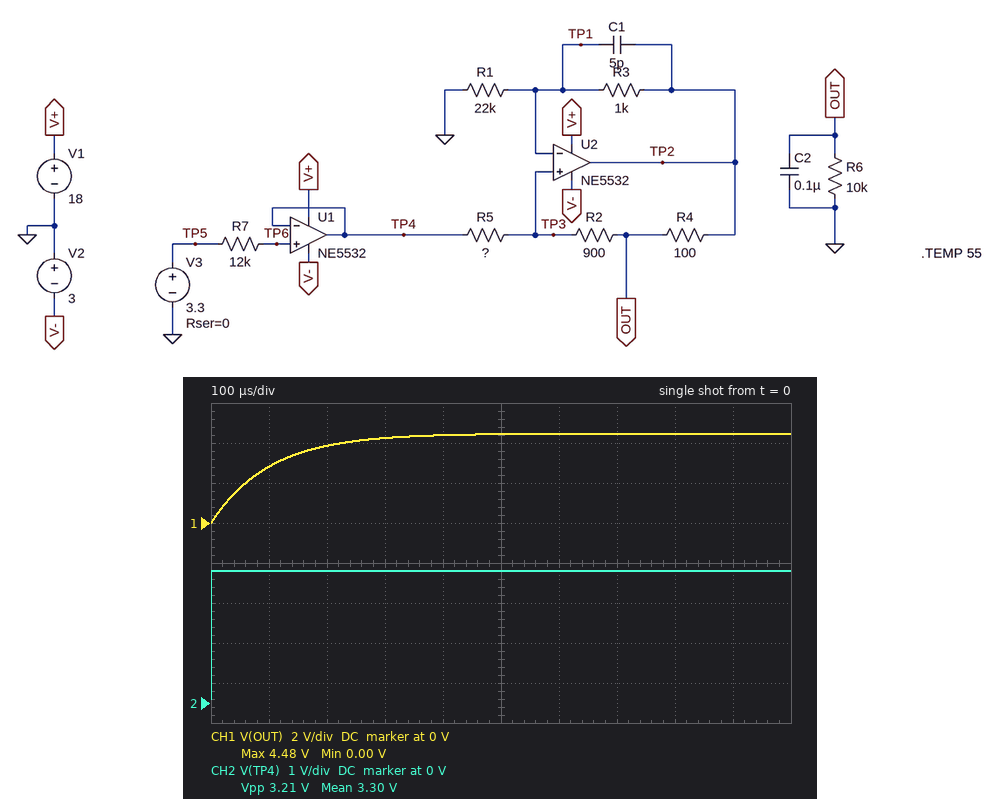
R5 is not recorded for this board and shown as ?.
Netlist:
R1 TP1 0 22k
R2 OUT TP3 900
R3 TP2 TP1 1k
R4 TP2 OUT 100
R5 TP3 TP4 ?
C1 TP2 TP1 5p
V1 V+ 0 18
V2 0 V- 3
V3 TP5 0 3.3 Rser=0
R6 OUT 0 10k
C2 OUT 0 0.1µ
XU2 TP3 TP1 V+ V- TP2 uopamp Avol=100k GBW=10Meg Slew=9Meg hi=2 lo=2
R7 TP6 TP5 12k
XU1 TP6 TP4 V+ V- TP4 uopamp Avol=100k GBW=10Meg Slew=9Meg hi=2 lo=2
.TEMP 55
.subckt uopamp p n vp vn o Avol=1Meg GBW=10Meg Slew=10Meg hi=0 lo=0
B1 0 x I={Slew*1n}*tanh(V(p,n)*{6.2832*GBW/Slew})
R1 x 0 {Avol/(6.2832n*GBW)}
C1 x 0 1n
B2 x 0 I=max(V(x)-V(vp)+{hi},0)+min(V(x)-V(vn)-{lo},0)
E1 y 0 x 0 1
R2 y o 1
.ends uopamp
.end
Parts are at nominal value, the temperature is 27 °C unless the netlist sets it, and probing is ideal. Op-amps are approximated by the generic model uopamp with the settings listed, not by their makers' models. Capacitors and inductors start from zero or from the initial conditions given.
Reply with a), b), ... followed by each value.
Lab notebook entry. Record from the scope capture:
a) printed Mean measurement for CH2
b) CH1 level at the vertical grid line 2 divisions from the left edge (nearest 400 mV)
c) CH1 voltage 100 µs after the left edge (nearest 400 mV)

a) 3.30 V
b) 4.0 V
c) 2.8 V
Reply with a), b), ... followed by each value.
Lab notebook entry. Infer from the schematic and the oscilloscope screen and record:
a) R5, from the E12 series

a) 6.8 kΩ
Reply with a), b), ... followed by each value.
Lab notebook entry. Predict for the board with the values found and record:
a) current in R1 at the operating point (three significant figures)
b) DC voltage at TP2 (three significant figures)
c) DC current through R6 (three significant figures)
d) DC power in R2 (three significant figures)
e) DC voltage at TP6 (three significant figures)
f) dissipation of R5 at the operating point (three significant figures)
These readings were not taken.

a) 197 µA
b) 4.53 V
c) 447 µA
d) 20.9 µW
e) 3.30 V
f) 158 µW
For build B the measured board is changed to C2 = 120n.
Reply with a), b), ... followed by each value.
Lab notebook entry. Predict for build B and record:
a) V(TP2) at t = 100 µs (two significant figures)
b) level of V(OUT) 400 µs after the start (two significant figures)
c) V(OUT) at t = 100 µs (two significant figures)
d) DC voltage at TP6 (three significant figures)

a) 2.7 V
b) 4.3 V
c) 2.5 V
d) 3.30 V
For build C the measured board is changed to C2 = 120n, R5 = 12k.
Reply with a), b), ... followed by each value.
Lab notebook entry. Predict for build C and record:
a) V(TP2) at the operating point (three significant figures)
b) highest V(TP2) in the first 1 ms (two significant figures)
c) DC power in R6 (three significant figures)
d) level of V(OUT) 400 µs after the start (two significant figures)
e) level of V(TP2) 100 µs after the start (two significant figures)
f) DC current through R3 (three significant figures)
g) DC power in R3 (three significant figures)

a) 5.96 V
b) 5.8 V
c) 3.46 mW
d) 4.6 V
e) 2.0 V
f) 259 µA
g) 67.2 µW
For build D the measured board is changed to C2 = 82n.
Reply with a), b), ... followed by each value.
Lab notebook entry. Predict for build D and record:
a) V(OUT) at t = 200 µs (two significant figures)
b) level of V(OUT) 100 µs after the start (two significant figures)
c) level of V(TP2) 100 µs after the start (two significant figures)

a) 4.1 V
b) 3.1 V
c) 3.3 V
